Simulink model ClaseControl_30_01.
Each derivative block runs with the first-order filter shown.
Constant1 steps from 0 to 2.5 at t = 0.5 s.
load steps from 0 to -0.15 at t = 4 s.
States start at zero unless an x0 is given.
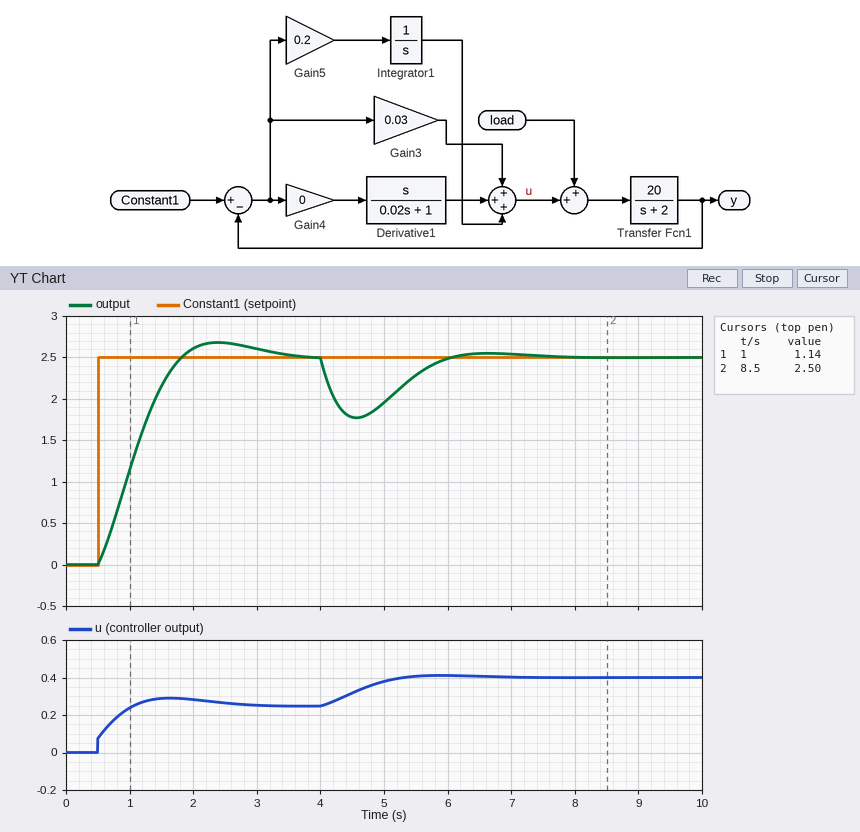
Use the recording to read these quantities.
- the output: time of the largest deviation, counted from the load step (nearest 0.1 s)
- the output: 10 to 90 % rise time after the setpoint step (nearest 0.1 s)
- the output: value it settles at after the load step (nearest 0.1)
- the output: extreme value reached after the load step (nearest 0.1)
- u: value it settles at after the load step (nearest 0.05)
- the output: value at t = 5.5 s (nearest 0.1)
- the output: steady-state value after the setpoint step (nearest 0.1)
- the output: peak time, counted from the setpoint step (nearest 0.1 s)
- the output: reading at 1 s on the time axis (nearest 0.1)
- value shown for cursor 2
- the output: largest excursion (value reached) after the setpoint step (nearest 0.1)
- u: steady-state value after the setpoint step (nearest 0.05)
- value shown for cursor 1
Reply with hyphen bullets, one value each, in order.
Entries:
- 0.6 s
- 0.9 s
- 2.5
- 1.8
- 0.40
- 2.3
- 2.5
- 1.9 s
- 1.1
- 2.50
- 2.7
- 0.25
- 1.14
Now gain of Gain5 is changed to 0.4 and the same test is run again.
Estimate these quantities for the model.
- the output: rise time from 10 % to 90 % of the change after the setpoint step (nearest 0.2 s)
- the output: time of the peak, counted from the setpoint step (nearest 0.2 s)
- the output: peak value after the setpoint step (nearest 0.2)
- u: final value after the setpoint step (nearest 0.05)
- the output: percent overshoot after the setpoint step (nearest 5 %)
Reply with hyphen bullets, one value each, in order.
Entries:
- 0.6 s
- 1.2 s
- 3.0
- 0.25
- 20 %
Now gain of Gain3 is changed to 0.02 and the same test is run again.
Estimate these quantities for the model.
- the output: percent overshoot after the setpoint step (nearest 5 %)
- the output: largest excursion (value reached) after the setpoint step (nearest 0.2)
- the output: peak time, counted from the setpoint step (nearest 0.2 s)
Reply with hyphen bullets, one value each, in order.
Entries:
- 10 %
- 2.8
- 1.8 s
